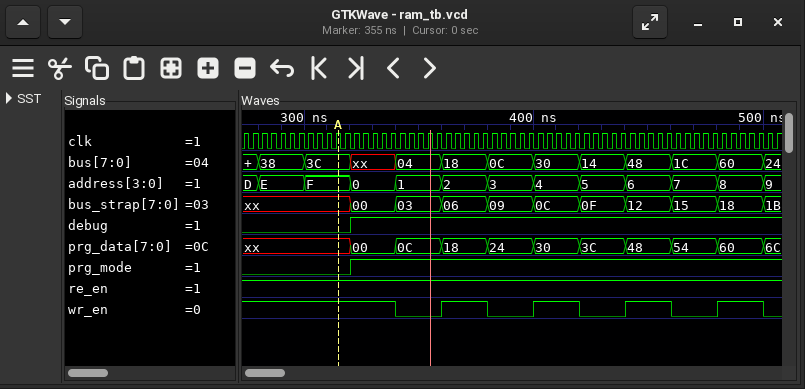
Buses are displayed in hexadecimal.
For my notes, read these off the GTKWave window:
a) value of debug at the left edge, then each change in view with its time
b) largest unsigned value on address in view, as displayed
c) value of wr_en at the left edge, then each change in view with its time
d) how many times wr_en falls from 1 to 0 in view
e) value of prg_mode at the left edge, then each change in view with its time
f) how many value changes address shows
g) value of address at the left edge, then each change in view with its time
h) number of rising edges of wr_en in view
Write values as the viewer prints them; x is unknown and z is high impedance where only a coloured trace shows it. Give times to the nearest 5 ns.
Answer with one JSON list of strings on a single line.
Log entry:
["0, 1 at 320 ns", "F", "1, 0 at 340 ns, 1 at 360 ns, 0 at 380 ns, 1 at 400 ns, 0 at 420 ns, 1 at 440 ns, 0 at 460 ns, 1 at 480 ns, 0 at 500 ns", "5", "0, 1 at 320 ns", "12", "D, E at 280 ns, F at 300 ns, 0 at 320 ns, 1 at 340 ns, 2 at 360 ns, 3 at 380 ns, 4 at 400 ns, 5 at 420 ns, 6 at 440 ns, 7 at 460 ns, 8 at 480 ns, 9 at 500 ns", "4"]
